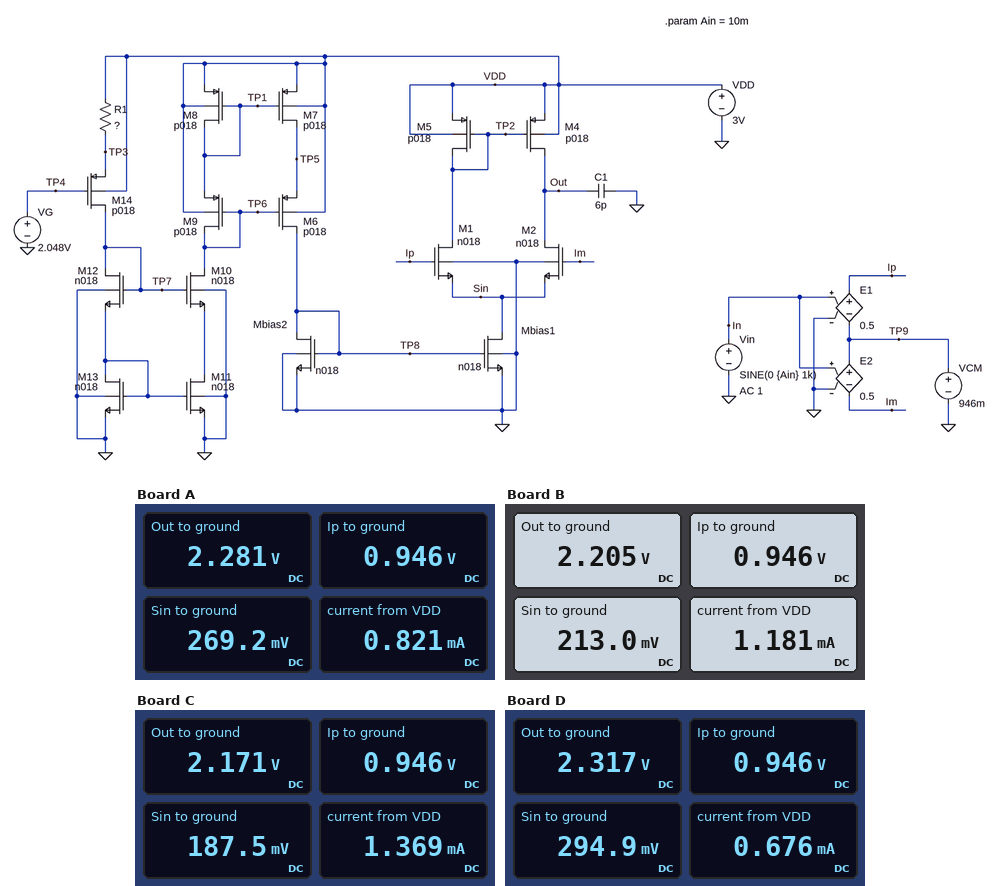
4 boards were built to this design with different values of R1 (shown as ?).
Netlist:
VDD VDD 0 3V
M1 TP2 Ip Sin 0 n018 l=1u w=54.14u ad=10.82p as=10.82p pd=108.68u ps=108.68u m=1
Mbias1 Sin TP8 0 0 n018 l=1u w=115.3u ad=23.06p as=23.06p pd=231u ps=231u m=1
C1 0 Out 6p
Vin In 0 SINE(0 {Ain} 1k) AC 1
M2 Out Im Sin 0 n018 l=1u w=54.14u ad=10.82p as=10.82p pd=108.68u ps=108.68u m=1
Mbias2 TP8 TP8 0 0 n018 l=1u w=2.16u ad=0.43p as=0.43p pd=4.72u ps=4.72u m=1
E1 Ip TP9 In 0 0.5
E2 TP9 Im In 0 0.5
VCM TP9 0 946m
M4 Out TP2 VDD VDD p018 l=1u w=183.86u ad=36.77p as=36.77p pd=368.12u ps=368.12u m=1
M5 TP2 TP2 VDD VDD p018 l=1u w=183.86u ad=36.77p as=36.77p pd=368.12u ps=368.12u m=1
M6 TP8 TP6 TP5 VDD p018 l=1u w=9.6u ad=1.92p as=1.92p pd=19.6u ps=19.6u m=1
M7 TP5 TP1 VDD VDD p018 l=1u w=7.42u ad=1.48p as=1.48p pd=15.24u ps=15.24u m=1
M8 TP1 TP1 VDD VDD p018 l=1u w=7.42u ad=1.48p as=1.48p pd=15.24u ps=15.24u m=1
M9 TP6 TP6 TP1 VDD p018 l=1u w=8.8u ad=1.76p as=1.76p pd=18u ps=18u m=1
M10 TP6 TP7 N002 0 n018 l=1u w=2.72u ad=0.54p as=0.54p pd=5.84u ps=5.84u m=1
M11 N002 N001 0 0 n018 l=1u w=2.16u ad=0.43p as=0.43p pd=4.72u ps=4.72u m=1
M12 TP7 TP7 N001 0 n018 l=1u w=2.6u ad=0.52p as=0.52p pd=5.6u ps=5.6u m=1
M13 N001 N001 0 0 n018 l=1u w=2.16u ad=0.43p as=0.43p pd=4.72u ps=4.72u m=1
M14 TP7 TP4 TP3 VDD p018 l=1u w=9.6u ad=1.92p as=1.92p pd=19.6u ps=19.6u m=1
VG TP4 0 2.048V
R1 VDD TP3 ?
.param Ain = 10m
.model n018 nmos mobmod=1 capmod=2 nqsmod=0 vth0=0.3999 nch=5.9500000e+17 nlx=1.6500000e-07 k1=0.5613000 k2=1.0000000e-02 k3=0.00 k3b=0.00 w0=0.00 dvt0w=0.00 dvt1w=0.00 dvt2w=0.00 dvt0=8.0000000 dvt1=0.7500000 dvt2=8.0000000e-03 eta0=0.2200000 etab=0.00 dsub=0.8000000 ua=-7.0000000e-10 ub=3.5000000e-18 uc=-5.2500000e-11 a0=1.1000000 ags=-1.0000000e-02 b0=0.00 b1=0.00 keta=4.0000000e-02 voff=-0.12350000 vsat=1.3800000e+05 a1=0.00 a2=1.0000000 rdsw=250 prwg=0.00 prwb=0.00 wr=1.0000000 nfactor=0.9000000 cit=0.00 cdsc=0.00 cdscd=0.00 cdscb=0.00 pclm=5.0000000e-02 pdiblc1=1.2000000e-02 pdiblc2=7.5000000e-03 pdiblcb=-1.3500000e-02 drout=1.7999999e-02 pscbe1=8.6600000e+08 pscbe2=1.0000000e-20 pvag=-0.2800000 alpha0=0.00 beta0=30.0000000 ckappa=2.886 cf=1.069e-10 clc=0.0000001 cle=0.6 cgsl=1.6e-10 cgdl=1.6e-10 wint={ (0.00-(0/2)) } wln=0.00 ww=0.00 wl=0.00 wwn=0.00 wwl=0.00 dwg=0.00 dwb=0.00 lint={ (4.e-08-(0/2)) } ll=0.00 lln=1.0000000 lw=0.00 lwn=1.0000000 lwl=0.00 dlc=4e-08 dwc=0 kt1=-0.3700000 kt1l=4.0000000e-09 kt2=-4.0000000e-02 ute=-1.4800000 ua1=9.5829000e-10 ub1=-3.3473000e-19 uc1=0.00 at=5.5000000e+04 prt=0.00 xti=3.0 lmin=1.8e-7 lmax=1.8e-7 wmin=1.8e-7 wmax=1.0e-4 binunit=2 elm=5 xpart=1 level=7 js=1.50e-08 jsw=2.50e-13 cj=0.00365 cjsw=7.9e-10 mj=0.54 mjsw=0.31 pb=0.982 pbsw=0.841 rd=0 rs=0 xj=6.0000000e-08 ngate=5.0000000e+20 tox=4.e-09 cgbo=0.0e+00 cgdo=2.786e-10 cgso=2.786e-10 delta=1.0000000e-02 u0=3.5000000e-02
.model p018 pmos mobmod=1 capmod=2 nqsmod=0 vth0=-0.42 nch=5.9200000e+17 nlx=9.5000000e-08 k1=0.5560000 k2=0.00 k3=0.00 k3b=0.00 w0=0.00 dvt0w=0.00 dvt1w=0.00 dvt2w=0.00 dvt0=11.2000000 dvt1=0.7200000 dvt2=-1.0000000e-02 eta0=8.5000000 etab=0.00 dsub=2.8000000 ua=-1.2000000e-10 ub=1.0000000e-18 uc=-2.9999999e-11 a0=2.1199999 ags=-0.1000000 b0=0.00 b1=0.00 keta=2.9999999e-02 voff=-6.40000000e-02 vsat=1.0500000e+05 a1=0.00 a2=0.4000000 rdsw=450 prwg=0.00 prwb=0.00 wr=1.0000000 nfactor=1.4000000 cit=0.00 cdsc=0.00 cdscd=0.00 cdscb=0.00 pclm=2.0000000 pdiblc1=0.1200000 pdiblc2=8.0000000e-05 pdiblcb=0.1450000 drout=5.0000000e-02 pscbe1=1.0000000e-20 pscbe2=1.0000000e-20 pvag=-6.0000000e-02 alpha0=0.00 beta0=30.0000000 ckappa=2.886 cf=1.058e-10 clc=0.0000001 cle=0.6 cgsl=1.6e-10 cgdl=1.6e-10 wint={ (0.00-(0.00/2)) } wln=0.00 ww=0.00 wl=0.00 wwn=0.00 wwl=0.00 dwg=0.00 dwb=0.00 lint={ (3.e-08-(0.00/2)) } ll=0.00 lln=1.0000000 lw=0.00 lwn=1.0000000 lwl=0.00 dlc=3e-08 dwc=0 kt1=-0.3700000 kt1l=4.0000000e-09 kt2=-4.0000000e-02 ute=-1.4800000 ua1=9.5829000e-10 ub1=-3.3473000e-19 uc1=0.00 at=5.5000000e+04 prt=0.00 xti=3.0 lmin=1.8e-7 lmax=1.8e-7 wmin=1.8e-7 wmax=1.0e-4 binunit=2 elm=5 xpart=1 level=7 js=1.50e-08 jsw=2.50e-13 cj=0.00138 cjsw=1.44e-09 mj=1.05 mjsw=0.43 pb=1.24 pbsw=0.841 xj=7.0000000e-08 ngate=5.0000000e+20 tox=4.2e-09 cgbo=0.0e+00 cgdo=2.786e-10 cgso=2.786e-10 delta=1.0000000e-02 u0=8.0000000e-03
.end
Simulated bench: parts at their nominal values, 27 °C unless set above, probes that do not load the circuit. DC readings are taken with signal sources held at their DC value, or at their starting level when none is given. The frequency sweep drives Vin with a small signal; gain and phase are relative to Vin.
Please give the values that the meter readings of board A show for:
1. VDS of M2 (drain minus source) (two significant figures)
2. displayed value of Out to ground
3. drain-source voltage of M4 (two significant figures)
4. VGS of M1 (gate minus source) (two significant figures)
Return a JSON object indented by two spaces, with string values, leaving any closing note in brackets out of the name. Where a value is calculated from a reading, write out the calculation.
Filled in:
{
  "VDS of M2 (drain minus source)": "2.281 V - 269.2 mV = 2.0 V",
  "displayed value of Out to ground": "2.281 V",
  "drain-source voltage of M4": "2.281 V - 3 V = -720 mV",
  "VGS of M1 (gate minus source)": "946 mV - 269.2 mV = 680 mV"
}
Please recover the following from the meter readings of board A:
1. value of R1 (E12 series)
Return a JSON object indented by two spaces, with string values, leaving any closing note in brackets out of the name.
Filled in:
{
  "value of R1": "27 kΩ"
}
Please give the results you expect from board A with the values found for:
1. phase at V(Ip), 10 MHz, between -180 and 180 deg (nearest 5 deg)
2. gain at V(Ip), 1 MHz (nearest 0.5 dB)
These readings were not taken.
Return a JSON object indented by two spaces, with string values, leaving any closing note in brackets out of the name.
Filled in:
{
  "phase at V(Ip), 10 MHz, between -180 and 180 deg": "0 deg",
  "gain at V(Ip), 1 MHz": "-6.0 dB"
}
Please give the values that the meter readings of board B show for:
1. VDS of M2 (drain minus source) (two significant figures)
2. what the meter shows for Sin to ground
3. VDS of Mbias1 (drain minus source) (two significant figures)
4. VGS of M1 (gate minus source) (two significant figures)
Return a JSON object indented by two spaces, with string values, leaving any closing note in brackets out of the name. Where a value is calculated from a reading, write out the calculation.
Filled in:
{
  "VDS of M2 (drain minus source)": "2.205 V - 213 mV = 2.0 V",
  "what the meter shows for Sin to ground": "213.0 mV",
  "VDS of Mbias1 (drain minus source)": "213 mV = 210 mV",
  "VGS of M1 (gate minus source)": "946 mV - 213 mV = 730 mV"
}
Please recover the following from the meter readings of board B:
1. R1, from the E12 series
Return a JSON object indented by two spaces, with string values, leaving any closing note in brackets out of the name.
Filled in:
{
  "R1, from the E12 series": "10 kΩ"
}
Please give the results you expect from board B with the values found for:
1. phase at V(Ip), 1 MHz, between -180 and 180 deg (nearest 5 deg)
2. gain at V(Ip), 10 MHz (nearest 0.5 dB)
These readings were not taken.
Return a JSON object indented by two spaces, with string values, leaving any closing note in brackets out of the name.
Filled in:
{
  "phase at V(Ip), 1 MHz, between -180 and 180 deg": "0 deg",
  "gain at V(Ip), 10 MHz": "-6.0 dB"
}
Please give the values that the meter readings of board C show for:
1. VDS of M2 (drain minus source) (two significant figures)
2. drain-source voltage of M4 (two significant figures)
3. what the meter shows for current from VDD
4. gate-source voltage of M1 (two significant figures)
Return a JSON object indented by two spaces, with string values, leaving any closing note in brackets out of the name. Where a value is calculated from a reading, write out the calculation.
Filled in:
{
  "VDS of M2 (drain minus source)": "2.171 V - 187.5 mV = 2.0 V",
  "drain-source voltage of M4": "2.171 V - 3 V = -830 mV",
  "what the meter shows for current from VDD": "1.369 mA",
  "gate-source voltage of M1": "946 mV - 187.5 mV = 760 mV"
}
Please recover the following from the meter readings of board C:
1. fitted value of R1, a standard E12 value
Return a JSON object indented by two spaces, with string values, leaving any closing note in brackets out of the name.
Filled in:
{
  "fitted value of R1, a standard E12 value": "4.7 kΩ"
}
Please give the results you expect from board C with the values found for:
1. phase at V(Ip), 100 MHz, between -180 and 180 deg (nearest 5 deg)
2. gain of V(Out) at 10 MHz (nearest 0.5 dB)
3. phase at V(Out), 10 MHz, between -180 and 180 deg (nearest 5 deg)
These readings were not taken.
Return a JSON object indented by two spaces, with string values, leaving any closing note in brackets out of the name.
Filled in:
{
  "phase at V(Ip), 100 MHz, between -180 and 180 deg": "0 deg",
  "gain of V(Out) at 10 MHz": "16.5 dB",
  "phase at V(Out), 10 MHz, between -180 and 180 deg": "-80 deg"
}
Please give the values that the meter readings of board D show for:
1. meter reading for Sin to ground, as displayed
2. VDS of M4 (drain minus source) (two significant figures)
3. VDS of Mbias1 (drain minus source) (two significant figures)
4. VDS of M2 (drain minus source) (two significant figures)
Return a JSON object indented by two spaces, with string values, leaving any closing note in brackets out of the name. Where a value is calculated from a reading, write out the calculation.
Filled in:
{
  "meter reading for Sin to ground, as displayed": "294.9 mV",
  "VDS of M4 (drain minus source)": "2.317 V - 3 V = -680 mV",
  "VDS of Mbias1 (drain minus source)": "294.9 mV = 290 mV",
  "VDS of M2 (drain minus source)": "2.317 V - 294.9 mV = 2.0 V"
}
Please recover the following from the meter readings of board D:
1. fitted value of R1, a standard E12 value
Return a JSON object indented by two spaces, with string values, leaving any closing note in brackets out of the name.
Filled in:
{
  "fitted value of R1, a standard E12 value": "39 kΩ"
}
